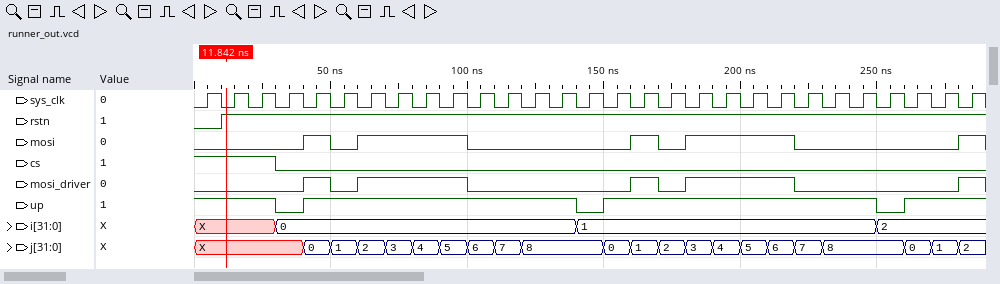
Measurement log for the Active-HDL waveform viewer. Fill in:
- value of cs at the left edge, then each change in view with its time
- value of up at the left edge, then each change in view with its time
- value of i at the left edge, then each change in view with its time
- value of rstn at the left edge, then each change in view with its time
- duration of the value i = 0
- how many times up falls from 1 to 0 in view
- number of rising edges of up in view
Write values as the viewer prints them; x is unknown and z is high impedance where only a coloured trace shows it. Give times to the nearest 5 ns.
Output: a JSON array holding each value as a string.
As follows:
["1, 0 at 30 ns", "1, 0 at 30 ns, 1 at 40 ns, 0 at 140 ns, 1 at 150 ns, 0 at 250 ns, 1 at 260 ns", "X, 0 at 30 ns, 1 at 140 ns, 2 at 250 ns", "0, 1 at 10 ns", "110 ns", "3", "3"]
